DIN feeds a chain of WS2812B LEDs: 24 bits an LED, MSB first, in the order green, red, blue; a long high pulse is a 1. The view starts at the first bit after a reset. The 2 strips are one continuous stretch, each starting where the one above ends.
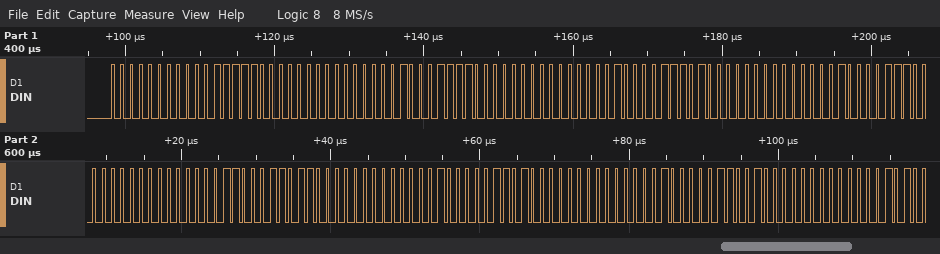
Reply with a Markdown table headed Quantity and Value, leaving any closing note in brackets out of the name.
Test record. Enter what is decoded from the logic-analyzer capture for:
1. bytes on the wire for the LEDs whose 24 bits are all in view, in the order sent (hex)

| Quantity | Value |
|---|---|
| bytes on the wire for the LEDs whose 24 bits are all in view, in the order sent | 00 1F 00 01 1E 00 02 1D 00 02 1C 00 03 1B 00 04 1A 00 04 19 00 |
